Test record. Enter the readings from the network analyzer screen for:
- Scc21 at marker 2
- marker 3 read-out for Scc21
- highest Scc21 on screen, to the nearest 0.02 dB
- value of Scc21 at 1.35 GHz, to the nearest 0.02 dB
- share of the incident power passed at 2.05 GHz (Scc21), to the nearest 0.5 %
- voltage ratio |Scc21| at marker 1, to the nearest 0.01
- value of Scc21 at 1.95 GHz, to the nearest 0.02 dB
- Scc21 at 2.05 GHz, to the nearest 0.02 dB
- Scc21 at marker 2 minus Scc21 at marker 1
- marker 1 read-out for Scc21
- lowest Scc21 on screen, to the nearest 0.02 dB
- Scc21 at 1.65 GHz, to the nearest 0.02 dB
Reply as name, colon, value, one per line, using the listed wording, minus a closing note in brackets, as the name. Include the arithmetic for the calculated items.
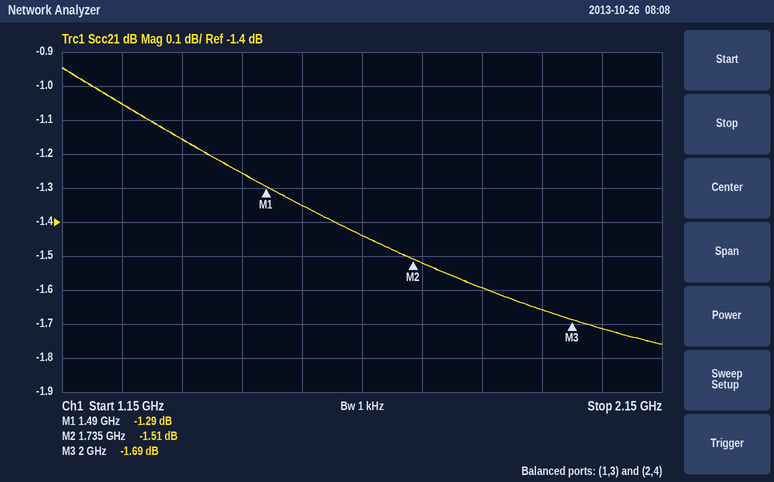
Scc21 at marker 2: -1.51 dB
marker 3 read-out for Scc21: -1.69 dB
highest Scc21 on screen, to the nearest 0.02 dB: -0.94 dB
value of Scc21 at 1.35 GHz, to the nearest 0.02 dB: -1.16 dB
share of the incident power passed at 2.05 GHz (Scc21), to the nearest 0.5 %: 10^(-1.72/10) ≈ 67.3 %, so 67.5 % to the nearest 0.5 %
voltage ratio |Scc21| at marker 1, to the nearest 0.01: 10^(-1.29/20) ≈ 0.86
value of Scc21 at 1.95 GHz, to the nearest 0.02 dB: -1.66 dB
Scc21 at 2.05 GHz, to the nearest 0.02 dB: -1.72 dB
Scc21 at marker 2 minus Scc21 at marker 1: -1.51 − (-1.29) = -0.22 dB
marker 1 read-out for Scc21: -1.29 dB
lowest Scc21 on screen, to the nearest 0.02 dB: -1.76 dB
Scc21 at 1.65 GHz, to the nearest 0.02 dB: -1.44 dB
